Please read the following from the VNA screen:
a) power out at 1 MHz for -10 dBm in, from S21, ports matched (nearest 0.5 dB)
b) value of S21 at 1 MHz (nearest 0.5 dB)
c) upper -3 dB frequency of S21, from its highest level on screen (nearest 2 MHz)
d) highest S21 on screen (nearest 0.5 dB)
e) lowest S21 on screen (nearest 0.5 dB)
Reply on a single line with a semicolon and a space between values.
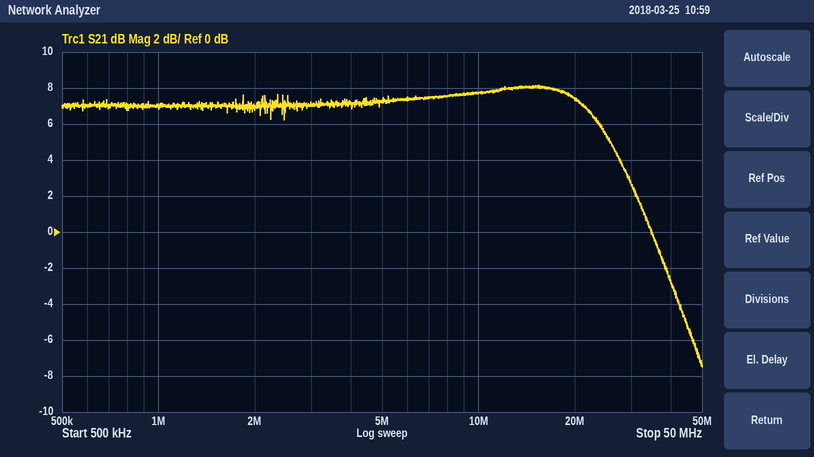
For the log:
-3.0 dBm; 7.0 dB; 26 MHz; 8.0 dB; -7.5 dB
